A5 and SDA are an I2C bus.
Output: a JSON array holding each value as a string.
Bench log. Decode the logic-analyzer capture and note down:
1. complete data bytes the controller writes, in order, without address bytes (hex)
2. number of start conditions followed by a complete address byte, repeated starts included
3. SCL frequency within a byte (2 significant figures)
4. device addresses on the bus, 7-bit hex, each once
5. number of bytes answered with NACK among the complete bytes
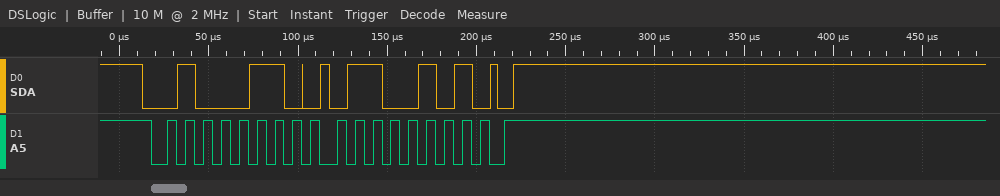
["65", "1", "100 kHz", "0x23", "0"]
